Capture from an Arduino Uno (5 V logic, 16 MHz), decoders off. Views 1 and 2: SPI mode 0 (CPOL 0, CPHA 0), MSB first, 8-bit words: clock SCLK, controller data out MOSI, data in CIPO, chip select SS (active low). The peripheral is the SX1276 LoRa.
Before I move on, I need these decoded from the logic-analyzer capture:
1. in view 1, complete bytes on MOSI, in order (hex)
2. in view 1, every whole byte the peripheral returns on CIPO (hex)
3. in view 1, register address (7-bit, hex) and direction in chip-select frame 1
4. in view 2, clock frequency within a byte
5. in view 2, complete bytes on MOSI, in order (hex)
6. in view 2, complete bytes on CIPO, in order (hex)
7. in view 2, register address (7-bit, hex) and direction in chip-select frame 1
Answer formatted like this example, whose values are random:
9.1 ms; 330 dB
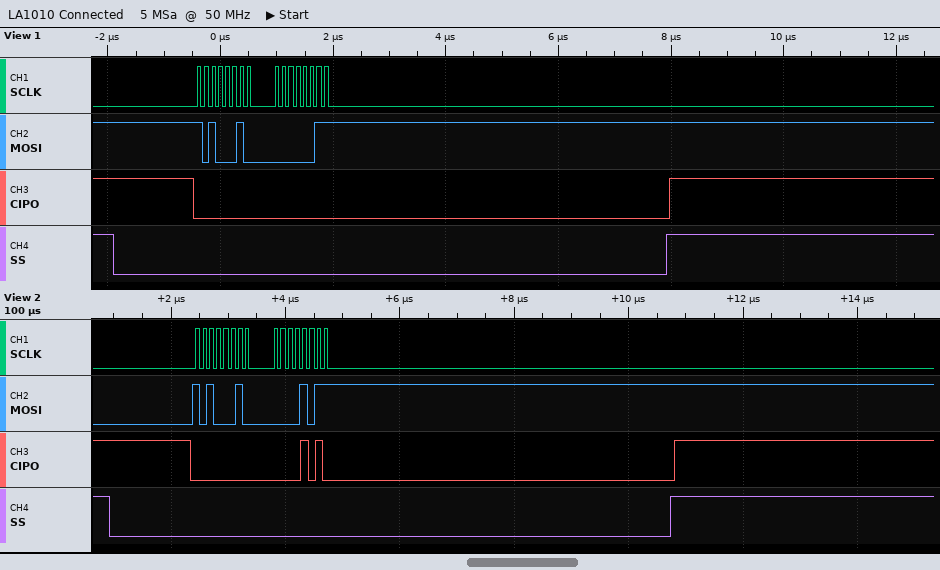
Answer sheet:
A2 03; 00 00; 0x22 write; 8 MHz; A2 0B; 00 0A; 0x22 write
